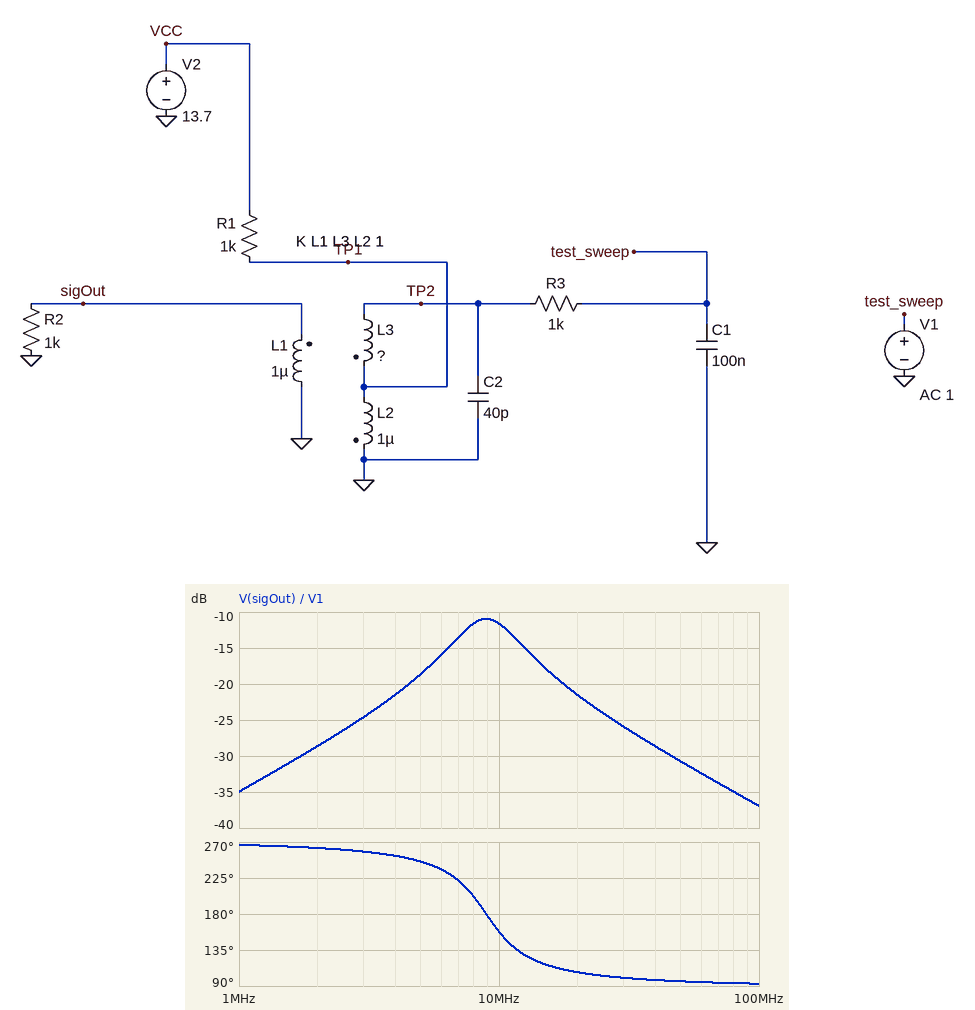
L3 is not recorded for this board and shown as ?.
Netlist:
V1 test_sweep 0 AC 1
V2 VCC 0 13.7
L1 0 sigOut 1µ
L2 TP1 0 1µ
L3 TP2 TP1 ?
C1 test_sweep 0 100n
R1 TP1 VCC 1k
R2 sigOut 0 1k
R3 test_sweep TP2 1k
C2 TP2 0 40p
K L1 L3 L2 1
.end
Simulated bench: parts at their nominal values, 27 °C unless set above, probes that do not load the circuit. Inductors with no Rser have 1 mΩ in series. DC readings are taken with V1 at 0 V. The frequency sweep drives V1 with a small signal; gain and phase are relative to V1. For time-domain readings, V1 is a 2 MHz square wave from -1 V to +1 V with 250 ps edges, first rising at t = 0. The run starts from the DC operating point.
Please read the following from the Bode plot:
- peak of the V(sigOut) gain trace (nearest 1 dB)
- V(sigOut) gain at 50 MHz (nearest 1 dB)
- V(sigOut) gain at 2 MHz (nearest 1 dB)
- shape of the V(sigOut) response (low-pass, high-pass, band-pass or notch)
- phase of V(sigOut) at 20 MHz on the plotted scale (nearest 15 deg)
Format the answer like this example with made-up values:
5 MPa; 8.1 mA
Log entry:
-11 dB; -31 dB; -29 dB; band-pass; 105 deg
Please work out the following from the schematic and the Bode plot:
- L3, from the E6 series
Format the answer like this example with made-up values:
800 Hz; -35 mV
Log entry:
3.3 µH
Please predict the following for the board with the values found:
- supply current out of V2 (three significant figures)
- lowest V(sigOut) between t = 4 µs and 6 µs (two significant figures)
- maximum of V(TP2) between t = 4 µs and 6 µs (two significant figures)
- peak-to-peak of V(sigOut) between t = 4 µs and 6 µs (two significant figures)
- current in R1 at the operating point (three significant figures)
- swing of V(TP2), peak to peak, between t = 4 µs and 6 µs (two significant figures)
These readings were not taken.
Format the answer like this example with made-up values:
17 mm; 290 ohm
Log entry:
13.7 mA; -210 mV; 600 mV; 430 mV; 13.7 mA; 1.2 V
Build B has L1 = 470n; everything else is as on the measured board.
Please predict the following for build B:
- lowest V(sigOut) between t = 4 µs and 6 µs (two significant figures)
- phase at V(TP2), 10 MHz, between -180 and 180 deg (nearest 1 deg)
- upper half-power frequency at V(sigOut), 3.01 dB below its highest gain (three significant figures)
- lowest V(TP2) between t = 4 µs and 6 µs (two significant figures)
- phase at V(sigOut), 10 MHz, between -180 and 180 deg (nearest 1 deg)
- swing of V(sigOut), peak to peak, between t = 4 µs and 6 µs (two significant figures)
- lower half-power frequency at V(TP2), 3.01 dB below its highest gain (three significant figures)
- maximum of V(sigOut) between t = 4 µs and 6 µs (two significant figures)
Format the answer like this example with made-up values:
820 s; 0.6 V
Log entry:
-150 mV; -23 deg; 11.6 MHz; -610 mV; 157 deg; 300 mV; 6.88 MHz; 150 mV
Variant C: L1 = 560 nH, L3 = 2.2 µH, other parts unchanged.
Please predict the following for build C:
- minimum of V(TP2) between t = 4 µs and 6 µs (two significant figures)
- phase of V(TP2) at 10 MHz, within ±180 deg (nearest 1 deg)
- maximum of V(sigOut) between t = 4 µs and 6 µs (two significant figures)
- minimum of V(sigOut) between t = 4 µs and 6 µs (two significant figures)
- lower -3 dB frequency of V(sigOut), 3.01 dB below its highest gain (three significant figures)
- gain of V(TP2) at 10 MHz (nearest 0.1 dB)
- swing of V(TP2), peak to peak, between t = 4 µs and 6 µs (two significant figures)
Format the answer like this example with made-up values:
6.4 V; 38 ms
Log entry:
-570 mV; 3 deg; 170 mV; -170 mV; 7.94 MHz; -2.0 dB; 1.1 V
